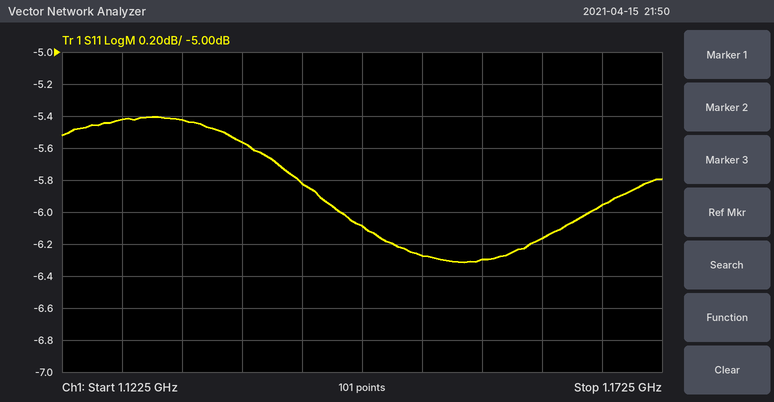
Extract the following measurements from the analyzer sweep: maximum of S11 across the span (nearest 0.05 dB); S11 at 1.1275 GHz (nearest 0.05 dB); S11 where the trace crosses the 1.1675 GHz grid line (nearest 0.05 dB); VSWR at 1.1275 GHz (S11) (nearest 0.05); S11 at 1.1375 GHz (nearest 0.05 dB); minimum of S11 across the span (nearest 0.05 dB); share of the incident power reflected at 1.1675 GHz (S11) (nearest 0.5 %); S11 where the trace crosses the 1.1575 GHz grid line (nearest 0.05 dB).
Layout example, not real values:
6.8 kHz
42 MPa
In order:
-5.40 dB
-5.40 dB
-5.95 dB
3.30
-5.55 dB
-6.30 dB
25.5 %
-6.30 dB
